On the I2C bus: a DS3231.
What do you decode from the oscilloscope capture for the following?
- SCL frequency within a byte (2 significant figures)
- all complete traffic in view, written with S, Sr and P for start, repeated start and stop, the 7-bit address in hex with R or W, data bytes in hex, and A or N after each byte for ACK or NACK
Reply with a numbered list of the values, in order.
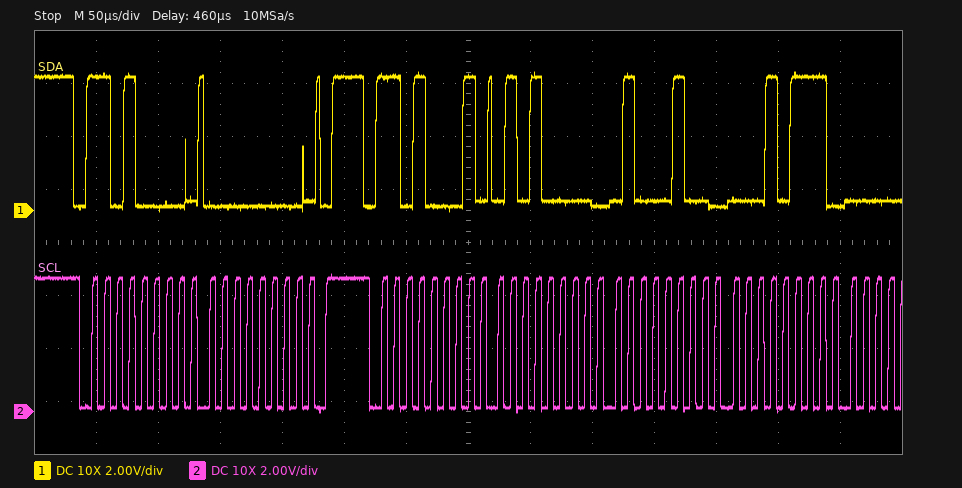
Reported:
1. 100 kHz
2. S 68W A 00 A P S 68R A 50 A 44 A 17 A
